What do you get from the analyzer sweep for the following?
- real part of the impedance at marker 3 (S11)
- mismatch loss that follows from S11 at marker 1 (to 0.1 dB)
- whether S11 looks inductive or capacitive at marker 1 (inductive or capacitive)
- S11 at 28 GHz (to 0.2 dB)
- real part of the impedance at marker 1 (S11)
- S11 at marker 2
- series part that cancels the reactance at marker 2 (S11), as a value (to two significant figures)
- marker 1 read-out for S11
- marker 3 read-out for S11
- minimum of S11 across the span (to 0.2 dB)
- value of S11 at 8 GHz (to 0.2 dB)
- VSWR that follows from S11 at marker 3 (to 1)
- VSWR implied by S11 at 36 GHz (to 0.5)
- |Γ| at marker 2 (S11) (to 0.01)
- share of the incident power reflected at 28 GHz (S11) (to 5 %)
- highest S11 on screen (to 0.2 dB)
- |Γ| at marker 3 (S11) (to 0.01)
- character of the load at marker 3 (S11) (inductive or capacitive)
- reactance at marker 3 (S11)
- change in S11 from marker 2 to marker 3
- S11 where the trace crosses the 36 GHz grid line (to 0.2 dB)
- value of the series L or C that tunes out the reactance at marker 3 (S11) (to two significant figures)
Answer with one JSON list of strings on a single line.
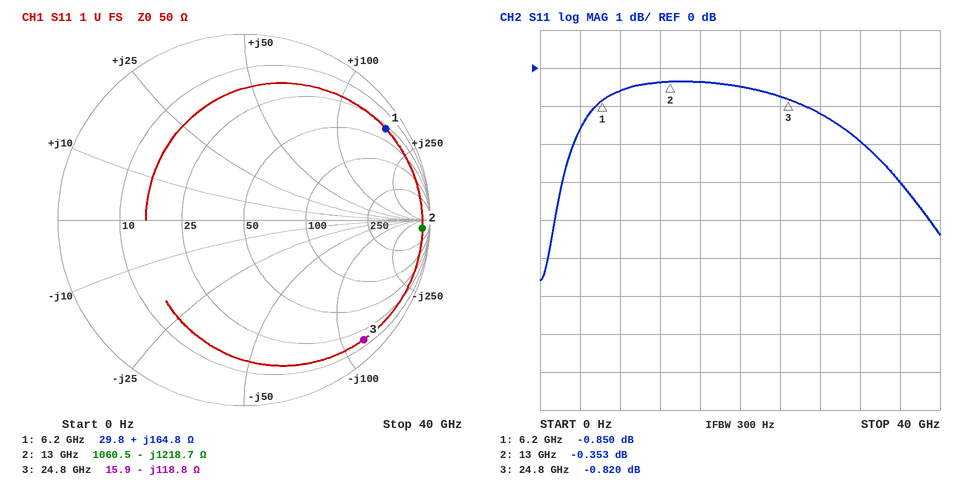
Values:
["15.9 Ω", "7.5 dB", "inductive", "-1.2 dB", "29.8 Ω", "-0.353 dB", "15 nH", "-0.850 dB", "-0.820 dB", "-5.6 dB", "-0.6 dB", "21", "6.0", "0.96", "75 %", "-0.4 dB", "0.91", "capacitive", "-118.8 Ω", "-0.467 dB", "-3.0 dB", "760 pH"]
